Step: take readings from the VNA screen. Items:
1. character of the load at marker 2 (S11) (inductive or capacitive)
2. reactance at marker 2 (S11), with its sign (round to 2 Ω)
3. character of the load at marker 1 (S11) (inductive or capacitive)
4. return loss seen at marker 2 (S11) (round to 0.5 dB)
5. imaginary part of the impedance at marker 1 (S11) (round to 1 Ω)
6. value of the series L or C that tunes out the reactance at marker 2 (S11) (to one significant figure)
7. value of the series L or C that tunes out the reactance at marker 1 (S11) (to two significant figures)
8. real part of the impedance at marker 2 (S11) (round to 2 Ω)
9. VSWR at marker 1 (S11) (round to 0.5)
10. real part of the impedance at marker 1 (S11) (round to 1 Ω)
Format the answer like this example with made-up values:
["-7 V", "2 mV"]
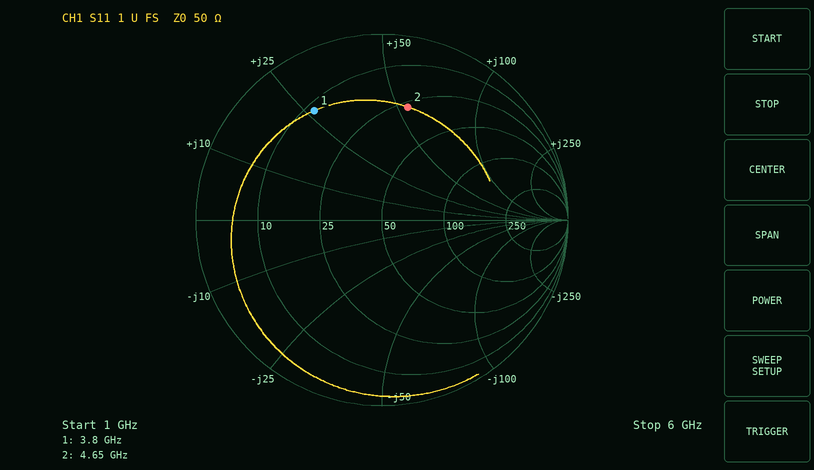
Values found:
["inductive", "+54 Ω", "inductive", "4.0 dB", "+27 Ω", "600 fF", "1.6 pF", "28 Ω", "5.5", "12 Ω"]
